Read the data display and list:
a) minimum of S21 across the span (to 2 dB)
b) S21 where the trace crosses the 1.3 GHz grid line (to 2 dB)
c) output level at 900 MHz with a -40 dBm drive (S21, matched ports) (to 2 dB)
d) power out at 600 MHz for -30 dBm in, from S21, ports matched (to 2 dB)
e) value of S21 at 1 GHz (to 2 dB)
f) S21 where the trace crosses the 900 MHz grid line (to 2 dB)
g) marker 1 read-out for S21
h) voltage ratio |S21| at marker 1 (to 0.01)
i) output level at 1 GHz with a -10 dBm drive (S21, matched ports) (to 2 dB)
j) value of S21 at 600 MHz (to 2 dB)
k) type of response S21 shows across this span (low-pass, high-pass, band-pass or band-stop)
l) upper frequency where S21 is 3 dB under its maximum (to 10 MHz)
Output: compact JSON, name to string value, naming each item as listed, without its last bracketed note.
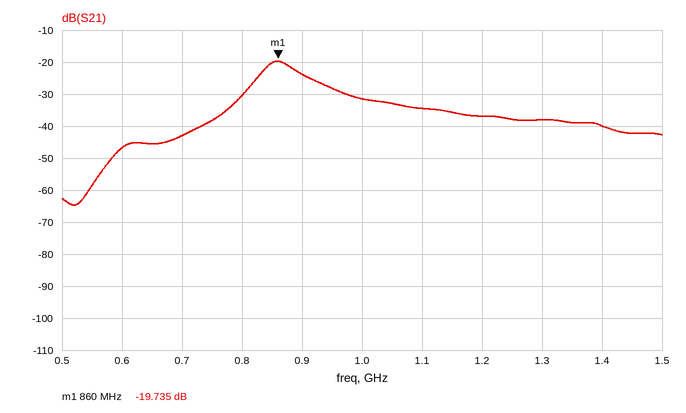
{"minimum of S21 across the span": "-64 dB", "S21 where the trace crosses the 1.3 GHz grid line": "-38 dB", "output level at 900 MHz with a -40 dBm drive (S21, matched ports)": "-64 dBm", "power out at 600 MHz for -30 dBm in, from S21, ports matched": "-76 dBm", "value of S21 at 1 GHz": "-32 dB", "S21 where the trace crosses the 900 MHz grid line": "-24 dB", "marker 1 read-out for S21": "-19.735 dB", "voltage ratio |S21| at marker 1": "0.10", "output level at 1 GHz with a -10 dBm drive (S21, matched ports)": "-42 dBm", "value of S21 at 600 MHz": "-46 dB", "type of response S21 shows across this span": "band-pass", "upper frequency where S21 is 3 dB under its maximum": "890 MHz"}
